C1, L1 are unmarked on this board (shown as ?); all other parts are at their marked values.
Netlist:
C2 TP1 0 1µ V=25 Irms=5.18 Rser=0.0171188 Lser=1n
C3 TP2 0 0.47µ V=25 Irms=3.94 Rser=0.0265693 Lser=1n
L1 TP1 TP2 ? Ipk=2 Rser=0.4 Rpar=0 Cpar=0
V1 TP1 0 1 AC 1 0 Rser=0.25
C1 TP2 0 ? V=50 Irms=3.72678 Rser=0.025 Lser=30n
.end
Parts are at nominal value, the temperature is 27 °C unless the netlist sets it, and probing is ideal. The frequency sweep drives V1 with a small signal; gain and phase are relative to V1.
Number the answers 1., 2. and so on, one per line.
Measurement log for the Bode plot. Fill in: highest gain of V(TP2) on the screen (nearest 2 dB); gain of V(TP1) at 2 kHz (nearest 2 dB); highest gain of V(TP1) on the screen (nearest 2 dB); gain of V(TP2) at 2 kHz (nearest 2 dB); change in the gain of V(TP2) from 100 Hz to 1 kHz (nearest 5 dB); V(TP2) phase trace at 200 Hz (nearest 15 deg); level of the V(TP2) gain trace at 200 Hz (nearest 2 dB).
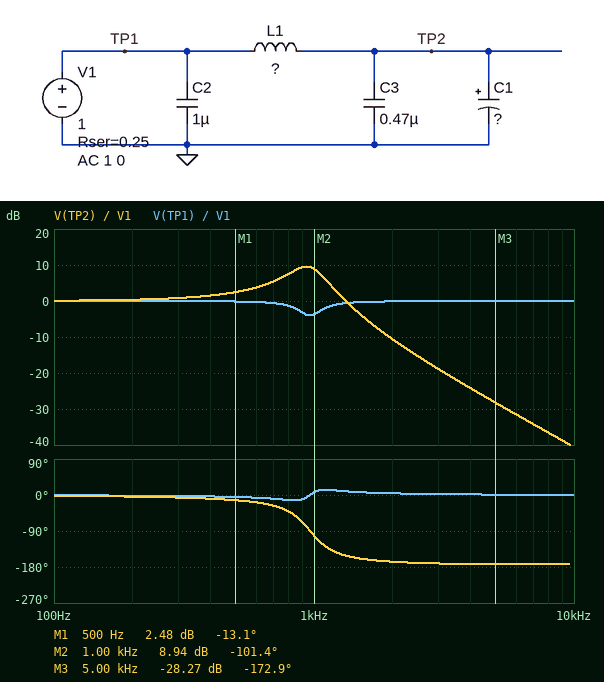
1. 10 dB
2. 0 dB
3. 0 dB
4. -10 dB
5. 10 dB
6. 0 deg
7. 0 dB
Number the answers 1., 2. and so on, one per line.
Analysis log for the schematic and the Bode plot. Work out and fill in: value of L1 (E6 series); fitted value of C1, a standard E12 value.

1. 330 µH
2. 82 µF
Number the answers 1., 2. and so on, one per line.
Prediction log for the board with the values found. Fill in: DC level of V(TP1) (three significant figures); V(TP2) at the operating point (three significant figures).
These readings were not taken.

1. 1.00 V
2. 1.00 V
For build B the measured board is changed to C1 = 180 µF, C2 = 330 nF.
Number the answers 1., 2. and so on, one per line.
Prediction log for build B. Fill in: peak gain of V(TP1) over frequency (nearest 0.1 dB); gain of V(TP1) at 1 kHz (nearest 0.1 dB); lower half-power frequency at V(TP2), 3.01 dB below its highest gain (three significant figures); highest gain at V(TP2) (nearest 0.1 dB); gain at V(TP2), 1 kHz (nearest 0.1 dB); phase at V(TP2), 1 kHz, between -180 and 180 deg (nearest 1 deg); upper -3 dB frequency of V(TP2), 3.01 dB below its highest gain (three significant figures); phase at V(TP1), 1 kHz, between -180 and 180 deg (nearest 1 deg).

1. 0 dB
2. -0.7 dB
3. 408 Hz
4. 6.3 dB
5. -3.8 dB
6. -149 deg
7. 760 Hz
8. 10 deg
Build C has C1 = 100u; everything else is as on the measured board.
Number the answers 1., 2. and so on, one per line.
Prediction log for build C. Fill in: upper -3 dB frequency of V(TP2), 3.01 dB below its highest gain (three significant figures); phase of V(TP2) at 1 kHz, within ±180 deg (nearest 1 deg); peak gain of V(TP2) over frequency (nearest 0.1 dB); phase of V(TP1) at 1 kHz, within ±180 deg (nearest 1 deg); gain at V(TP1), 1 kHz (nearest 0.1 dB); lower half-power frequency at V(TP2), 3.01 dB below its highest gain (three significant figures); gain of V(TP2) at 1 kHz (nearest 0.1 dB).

1. 995 Hz
2. -125 deg
3. 8.7 dB
4. 13 deg
5. -2.2 dB
6. 657 Hz
7. 5.6 dB
